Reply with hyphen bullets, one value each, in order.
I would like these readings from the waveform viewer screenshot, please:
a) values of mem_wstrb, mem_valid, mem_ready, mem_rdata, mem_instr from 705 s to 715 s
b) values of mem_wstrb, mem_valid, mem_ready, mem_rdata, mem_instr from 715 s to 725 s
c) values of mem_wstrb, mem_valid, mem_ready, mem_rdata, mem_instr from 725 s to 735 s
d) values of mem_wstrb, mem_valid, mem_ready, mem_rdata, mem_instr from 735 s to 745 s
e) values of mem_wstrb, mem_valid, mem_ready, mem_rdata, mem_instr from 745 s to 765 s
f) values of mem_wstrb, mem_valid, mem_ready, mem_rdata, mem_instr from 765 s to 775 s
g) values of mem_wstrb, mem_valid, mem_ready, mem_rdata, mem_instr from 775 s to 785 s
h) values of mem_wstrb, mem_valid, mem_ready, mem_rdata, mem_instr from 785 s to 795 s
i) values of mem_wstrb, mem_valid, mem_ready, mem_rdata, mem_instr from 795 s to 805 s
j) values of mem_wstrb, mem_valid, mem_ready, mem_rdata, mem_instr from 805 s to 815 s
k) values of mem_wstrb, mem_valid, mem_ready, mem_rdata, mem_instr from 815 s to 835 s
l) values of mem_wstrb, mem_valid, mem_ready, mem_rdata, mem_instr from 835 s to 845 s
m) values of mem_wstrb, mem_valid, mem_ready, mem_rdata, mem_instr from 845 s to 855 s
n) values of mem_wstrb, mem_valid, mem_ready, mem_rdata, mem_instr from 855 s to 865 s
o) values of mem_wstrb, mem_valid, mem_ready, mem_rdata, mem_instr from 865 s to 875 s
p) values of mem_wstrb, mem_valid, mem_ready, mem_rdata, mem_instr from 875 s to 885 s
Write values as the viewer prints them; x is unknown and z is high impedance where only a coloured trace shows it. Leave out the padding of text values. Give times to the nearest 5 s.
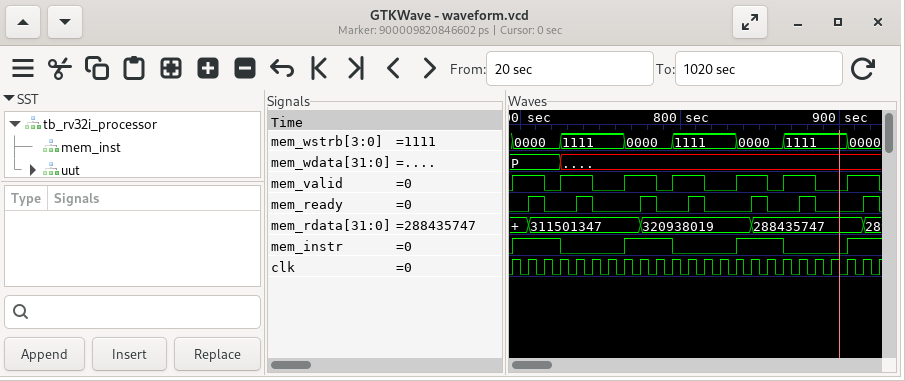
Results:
- mem_wstrb=0000, mem_valid=1, mem_ready=1, mem_rdata=311501347, mem_instr=1
- mem_wstrb=0000, mem_valid=0, mem_ready=0, mem_rdata=311501347, mem_instr=1
- mem_wstrb=1111, mem_valid=1, mem_ready=0, mem_rdata=311501347, mem_instr=0
- mem_wstrb=1111, mem_valid=1, mem_ready=1, mem_rdata=311501347, mem_instr=0
- mem_wstrb=1111, mem_valid=0, mem_ready=0, mem_rdata=311501347, mem_instr=0
- mem_wstrb=0000, mem_valid=1, mem_ready=0, mem_rdata=311501347, mem_instr=1
- mem_wstrb=0000, mem_valid=1, mem_ready=1, mem_rdata=320938019, mem_instr=1
- mem_wstrb=0000, mem_valid=0, mem_ready=0, mem_rdata=320938019, mem_instr=1
- mem_wstrb=1111, mem_valid=1, mem_ready=0, mem_rdata=320938019, mem_instr=0
- mem_wstrb=1111, mem_valid=1, mem_ready=1, mem_rdata=320938019, mem_instr=0
- mem_wstrb=1111, mem_valid=0, mem_ready=0, mem_rdata=320938019, mem_instr=0
- mem_wstrb=0000, mem_valid=1, mem_ready=0, mem_rdata=320938019, mem_instr=1
- mem_wstrb=0000, mem_valid=1, mem_ready=1, mem_rdata=288435747, mem_instr=1
- mem_wstrb=0000, mem_valid=0, mem_ready=0, mem_rdata=288435747, mem_instr=1
- mem_wstrb=1111, mem_valid=1, mem_ready=0, mem_rdata=288435747, mem_instr=0
- mem_wstrb=1111, mem_valid=1, mem_ready=1, mem_rdata=288435747, mem_instr=0
